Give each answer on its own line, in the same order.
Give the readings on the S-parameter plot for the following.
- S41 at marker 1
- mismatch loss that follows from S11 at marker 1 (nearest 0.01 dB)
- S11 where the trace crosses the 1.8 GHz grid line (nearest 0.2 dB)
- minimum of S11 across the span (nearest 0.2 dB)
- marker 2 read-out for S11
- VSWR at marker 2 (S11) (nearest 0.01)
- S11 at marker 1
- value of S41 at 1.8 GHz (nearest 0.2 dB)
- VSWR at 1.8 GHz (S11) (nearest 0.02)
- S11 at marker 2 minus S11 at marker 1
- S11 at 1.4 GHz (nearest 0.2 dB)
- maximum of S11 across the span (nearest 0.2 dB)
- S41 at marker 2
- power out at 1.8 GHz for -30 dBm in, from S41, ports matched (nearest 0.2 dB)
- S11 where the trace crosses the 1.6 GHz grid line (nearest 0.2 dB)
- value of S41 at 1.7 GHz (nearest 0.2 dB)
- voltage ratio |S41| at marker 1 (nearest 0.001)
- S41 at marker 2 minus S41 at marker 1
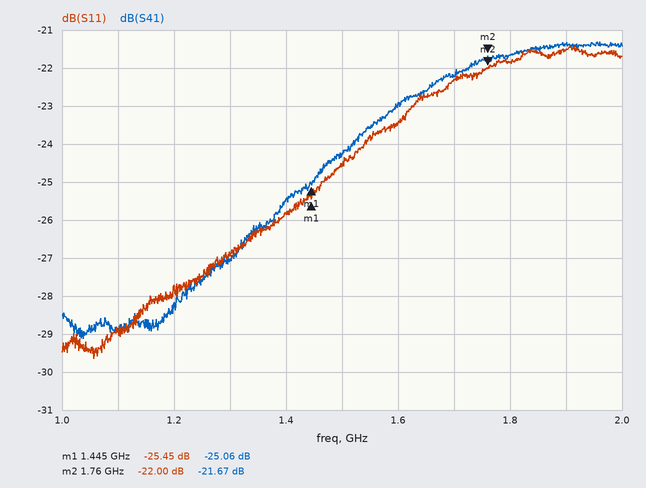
-25.06 dB
0.01 dB
-21.8 dB
-29.6 dB
-22.00 dB
1.17
-25.45 dB
-21.6 dB
1.18
3.45 dB
-25.8 dB
-21.4 dB
-21.67 dB
-51.6 dBm
-23.4 dB
-22.2 dB
0.056
3.39 dB
